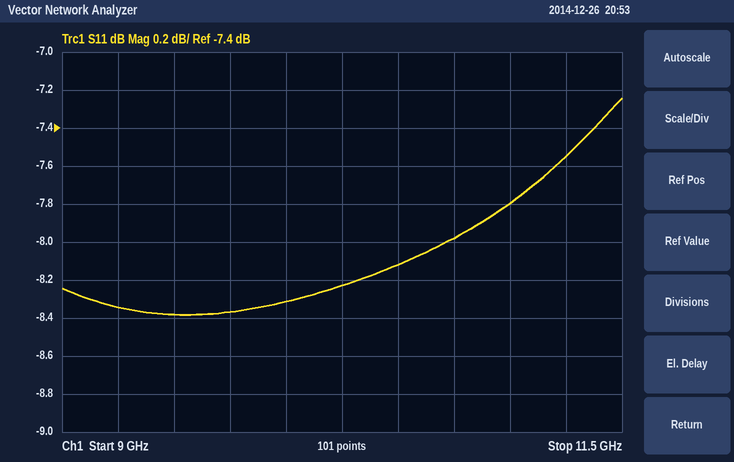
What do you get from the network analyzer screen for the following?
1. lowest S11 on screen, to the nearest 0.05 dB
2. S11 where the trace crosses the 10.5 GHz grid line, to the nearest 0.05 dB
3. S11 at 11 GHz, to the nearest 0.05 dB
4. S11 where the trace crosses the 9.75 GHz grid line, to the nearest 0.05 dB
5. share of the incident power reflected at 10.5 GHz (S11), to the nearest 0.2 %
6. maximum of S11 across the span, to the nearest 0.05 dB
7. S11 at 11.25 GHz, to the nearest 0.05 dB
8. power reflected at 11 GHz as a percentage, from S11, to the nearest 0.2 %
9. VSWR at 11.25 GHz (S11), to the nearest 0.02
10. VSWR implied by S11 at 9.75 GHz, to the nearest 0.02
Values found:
-8.40 dB
-8.10 dB
-7.80 dB
-8.35 dB
15.4 %
-7.25 dB
-7.55 dB
16.6 %
2.44
2.24
